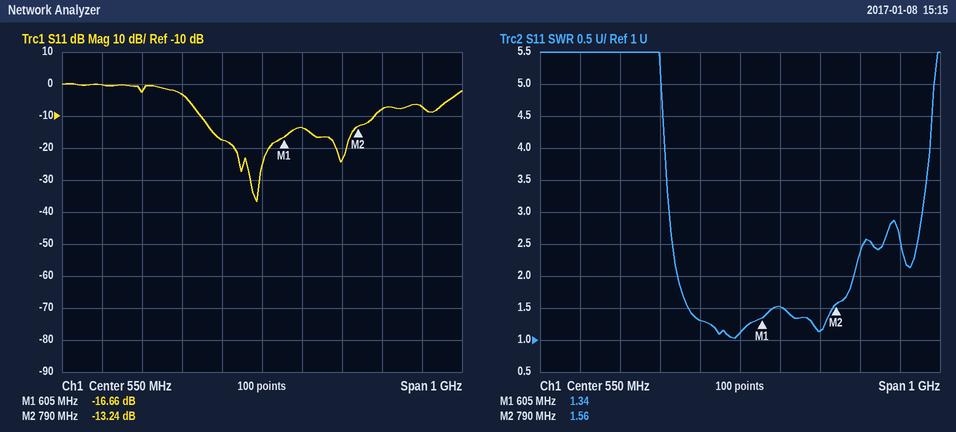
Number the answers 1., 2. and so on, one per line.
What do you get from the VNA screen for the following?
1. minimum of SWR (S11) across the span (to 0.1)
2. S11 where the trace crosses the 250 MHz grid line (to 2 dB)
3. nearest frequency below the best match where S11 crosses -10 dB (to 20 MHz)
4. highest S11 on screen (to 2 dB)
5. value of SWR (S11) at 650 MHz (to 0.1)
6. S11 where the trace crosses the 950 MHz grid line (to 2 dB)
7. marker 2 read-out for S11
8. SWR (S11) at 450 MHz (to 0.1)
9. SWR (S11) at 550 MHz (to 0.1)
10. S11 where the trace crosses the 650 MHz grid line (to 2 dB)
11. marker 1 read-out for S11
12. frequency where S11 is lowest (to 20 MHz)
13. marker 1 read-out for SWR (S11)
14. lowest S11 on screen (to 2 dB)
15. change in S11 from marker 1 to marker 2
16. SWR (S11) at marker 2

1. 1.0
2. -2 dB
3. 400 MHz
4. 0 dB
5. 1.5
6. -8 dB
7. -13.24 dB
8. 1.3
9. 1.1
10. -14 dB
11. -16.66 dB
12. 540 MHz
13. 1.34
14. -36 dB
15. 3.42 dB
16. 1.56
